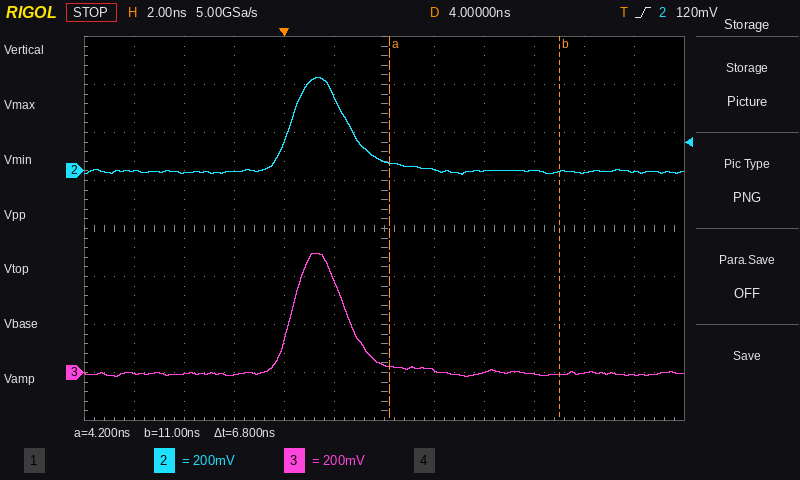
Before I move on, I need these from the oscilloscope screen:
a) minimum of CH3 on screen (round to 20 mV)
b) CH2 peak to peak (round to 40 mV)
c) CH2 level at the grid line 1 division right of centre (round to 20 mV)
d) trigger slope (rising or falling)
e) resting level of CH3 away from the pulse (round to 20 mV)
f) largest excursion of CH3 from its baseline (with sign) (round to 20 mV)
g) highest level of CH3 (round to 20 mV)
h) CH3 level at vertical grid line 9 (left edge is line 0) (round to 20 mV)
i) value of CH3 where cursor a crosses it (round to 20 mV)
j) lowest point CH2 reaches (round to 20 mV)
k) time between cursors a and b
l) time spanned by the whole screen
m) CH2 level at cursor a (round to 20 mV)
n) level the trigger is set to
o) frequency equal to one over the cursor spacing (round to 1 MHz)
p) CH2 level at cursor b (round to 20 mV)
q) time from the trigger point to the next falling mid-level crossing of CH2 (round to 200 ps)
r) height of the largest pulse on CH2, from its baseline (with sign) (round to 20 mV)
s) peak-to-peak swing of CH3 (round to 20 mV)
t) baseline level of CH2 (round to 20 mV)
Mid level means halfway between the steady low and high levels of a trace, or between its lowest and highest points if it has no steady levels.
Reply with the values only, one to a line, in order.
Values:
-20 mV
400 mV
0 mV
rising
0 mV
+500 mV
500 mV
0 mV
20 mV
-20 mV
6.8 ns
24 ns
40 mV
120 mV
147 MHz
0 mV
2.6 ns
+400 mV
520 mV
0 mV
